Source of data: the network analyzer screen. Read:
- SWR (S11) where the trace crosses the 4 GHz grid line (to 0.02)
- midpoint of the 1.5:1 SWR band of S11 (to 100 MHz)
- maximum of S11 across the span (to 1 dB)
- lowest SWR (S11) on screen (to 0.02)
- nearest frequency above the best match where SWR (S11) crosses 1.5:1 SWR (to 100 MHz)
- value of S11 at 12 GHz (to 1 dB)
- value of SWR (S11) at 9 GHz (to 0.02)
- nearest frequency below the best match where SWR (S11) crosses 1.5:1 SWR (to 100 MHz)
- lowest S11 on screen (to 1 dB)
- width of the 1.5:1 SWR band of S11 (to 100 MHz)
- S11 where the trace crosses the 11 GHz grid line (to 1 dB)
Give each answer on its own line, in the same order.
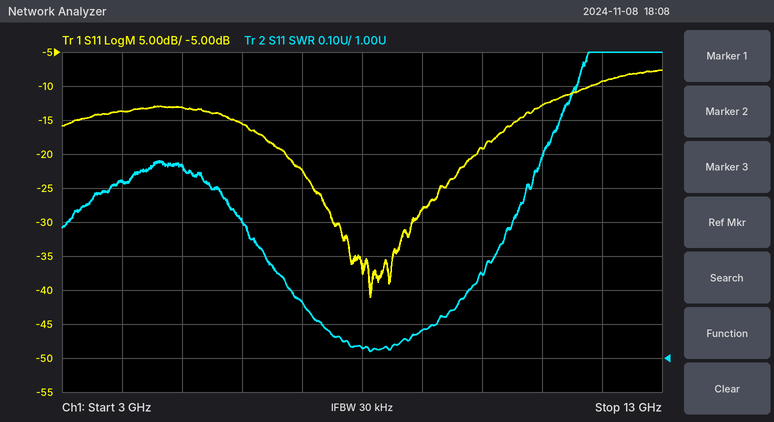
1.52
8.2 GHz
-8 dB
1.02
10.7 GHz
-9 dB
1.08
5.6 GHz
-41 dB
5.1 GHz
-13 dB
